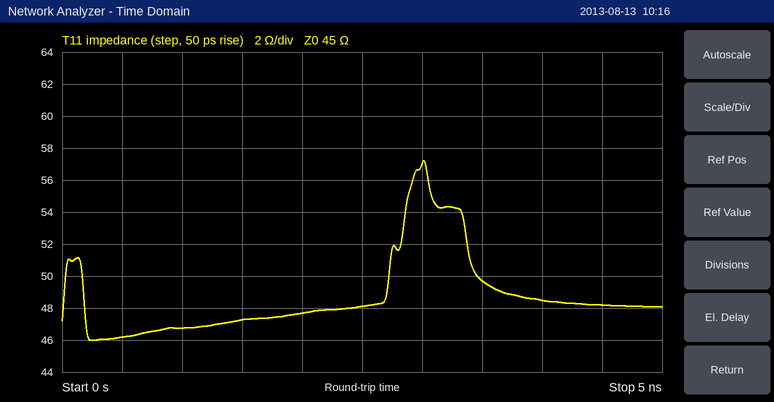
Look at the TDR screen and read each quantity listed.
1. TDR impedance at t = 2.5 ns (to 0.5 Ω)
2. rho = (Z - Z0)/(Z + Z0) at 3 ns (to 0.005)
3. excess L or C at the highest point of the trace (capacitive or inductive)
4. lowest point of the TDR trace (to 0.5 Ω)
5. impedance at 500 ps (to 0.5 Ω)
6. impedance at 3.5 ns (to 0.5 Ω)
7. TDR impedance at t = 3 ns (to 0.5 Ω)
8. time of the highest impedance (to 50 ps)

48.0 Ω
+0.120
inductive
46.0 Ω
46.0 Ω
49.5 Ω
57.0 Ω
3.00 ns
